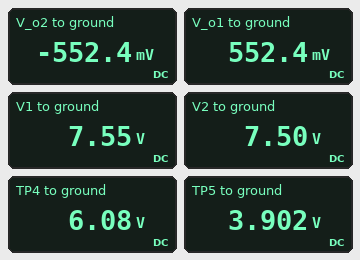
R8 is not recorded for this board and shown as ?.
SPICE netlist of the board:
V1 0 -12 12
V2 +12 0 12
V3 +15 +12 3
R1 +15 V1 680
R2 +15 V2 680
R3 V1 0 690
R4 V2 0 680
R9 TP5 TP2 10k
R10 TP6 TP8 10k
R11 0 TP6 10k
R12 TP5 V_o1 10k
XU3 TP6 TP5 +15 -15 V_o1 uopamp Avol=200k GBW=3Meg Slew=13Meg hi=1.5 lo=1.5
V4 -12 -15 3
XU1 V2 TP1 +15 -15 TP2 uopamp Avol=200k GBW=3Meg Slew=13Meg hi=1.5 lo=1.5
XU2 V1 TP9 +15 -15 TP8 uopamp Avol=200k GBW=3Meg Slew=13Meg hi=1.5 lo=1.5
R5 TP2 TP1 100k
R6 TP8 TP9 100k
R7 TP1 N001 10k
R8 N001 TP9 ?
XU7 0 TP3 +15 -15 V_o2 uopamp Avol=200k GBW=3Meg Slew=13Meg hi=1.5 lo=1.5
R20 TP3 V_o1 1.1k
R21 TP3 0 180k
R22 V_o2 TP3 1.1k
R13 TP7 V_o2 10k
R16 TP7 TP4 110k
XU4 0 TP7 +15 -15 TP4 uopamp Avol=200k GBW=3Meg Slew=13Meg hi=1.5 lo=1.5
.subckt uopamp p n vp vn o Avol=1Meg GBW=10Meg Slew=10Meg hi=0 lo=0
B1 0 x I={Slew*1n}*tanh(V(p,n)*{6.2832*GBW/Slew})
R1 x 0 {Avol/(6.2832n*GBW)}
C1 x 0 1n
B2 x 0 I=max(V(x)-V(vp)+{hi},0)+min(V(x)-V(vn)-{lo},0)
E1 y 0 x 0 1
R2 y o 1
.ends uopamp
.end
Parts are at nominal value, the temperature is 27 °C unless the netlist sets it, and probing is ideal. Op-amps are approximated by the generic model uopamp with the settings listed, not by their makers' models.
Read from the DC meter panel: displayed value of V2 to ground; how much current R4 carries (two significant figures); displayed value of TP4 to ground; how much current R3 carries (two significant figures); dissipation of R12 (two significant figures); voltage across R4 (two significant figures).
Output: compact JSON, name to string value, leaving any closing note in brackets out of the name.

{"displayed value of V2 to ground": "7.50 V", "how much current R4 carries": "11 mA", "displayed value of TP4 to ground": "6.08 V", "how much current R3 carries": "11 mA", "dissipation of R12": "1.1 mW", "voltage across R4": "7.5 V"}
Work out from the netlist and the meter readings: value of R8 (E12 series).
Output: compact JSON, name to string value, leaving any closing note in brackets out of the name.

{"value of R8": "12 kΩ"}
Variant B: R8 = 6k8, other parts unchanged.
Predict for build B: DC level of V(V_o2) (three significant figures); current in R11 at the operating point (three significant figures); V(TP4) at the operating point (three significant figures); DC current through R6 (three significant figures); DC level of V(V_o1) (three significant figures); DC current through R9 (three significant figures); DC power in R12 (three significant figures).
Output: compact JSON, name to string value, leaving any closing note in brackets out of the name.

{"DC level of V(V_o2)": "-706 mV", "current in R11 at the operating point": "394 µA", "V(TP4) at the operating point": "7.77 V", "DC current through R6": "3.26 µA", "DC level of V(V_o1)": "706 mV", "DC current through R9": "323 µA", "DC power in R12": "1.05 mW"}
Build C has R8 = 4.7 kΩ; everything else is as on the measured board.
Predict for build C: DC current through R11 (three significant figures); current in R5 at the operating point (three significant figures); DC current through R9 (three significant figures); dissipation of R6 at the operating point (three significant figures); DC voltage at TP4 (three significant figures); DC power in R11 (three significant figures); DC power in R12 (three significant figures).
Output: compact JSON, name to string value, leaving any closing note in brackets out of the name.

{"DC current through R11": "396 µA", "current in R5 at the operating point": "3.72 µA", "DC current through R9": "316 µA", "dissipation of R6 at the operating point": "1.39 µW", "DC voltage at TP4": "8.79 V", "DC power in R11": "1.57 mW", "DC power in R12": "1.00 mW"}
